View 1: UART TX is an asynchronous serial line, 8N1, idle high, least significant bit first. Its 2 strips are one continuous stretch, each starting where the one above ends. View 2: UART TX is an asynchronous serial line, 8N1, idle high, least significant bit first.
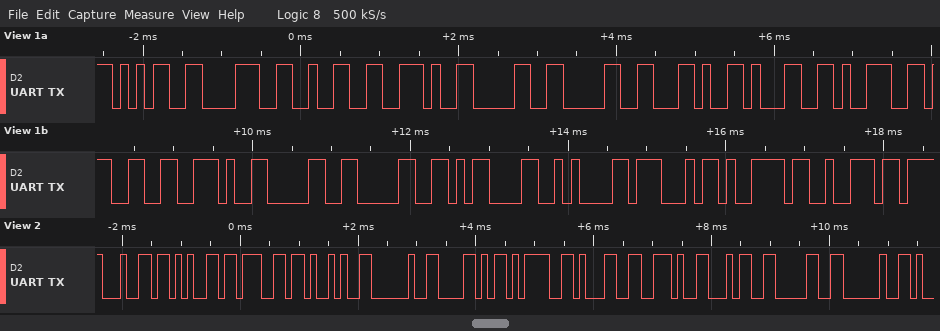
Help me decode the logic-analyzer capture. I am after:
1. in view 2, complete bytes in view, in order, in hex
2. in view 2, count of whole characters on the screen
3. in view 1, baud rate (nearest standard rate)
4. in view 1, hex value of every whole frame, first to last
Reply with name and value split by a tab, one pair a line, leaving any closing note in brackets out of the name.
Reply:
in view 2, complete bytes in view, in order, in hex	64 65 67 29 20 58 3D 31 2E 34 30 20
in view 2, count of whole characters on the screen	12
in view 1, baud rate	9600 baud
in view 1, hex value of every whole frame, first to last	0x35 0x38 0x32 0x2E 0x30 0x30 0x2C 0x31 0x39 0x33 0x2E 0x30 0x30 0x0D 0x0A 0x47 0x79 0x72
